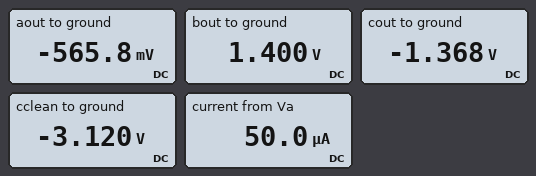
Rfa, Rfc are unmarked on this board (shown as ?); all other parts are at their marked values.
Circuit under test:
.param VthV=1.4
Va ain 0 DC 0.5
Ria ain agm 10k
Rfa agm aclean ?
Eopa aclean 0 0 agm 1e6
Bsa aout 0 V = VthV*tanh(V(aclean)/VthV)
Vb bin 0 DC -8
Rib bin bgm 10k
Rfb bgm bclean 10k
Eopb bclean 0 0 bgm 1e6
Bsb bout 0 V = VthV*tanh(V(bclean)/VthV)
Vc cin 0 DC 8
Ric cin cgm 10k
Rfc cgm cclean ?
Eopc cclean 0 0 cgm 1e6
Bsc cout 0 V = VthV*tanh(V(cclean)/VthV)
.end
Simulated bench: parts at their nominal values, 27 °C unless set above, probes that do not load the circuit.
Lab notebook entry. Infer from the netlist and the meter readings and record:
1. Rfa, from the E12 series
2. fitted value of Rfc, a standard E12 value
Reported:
12 kΩ
3.9 kΩ
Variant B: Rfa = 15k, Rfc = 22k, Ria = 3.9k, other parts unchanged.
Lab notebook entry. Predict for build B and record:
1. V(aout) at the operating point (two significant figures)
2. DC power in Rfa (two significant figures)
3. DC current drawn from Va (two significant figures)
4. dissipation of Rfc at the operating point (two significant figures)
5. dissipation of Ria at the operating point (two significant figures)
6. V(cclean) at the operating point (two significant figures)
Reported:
-1.2 V
250 µW
130 µA
14 mW
64 µW
-18 V
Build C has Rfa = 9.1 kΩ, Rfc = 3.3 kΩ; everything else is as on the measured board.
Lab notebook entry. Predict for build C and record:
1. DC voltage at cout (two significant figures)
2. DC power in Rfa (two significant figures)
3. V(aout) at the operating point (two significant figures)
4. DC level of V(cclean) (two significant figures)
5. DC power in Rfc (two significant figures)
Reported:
-1.3 V
23 µW
-440 mV
-2.6 V
2.1 mW
